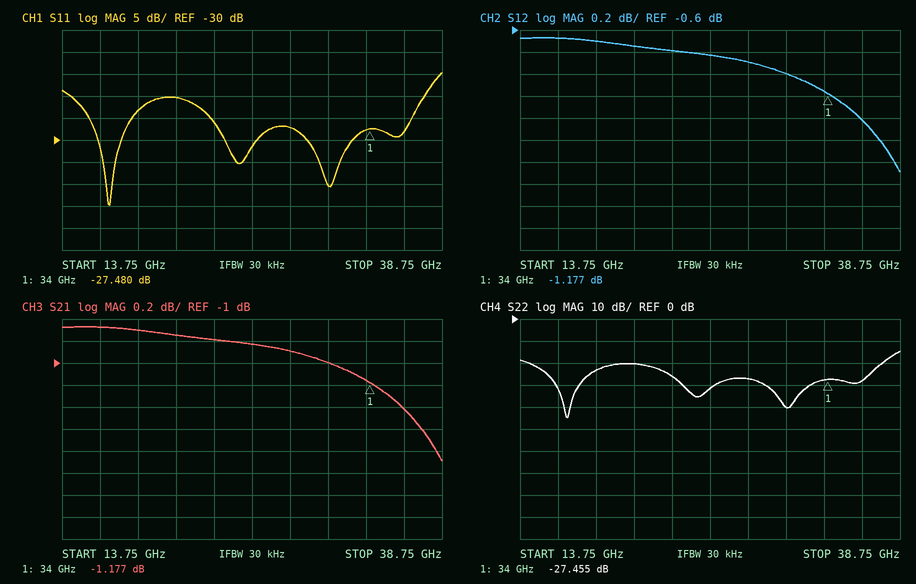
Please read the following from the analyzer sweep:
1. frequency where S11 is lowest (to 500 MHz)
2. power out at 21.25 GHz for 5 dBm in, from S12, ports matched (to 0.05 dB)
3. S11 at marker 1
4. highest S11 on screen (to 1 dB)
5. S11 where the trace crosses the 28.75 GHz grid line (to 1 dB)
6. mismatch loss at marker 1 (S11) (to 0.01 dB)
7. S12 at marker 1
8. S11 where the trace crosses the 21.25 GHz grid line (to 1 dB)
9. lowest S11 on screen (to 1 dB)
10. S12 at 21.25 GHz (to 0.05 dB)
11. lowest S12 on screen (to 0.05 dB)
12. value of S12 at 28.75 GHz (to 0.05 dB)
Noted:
17.0 GHz
4.25 dBm
-27.480 dB
-15 dB
-27 dB
0.01 dB
-1.177 dB
-20 dB
-45 dB
-0.75 dB
-1.90 dB
-0.90 dB
